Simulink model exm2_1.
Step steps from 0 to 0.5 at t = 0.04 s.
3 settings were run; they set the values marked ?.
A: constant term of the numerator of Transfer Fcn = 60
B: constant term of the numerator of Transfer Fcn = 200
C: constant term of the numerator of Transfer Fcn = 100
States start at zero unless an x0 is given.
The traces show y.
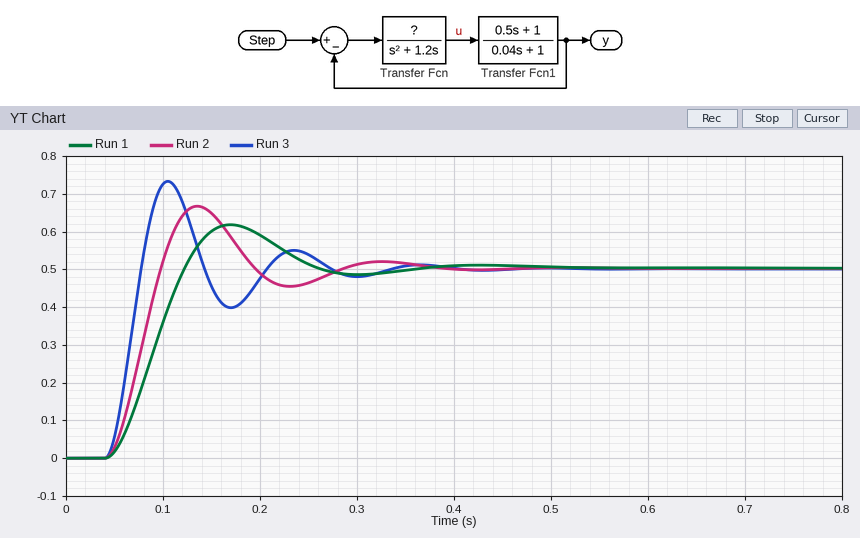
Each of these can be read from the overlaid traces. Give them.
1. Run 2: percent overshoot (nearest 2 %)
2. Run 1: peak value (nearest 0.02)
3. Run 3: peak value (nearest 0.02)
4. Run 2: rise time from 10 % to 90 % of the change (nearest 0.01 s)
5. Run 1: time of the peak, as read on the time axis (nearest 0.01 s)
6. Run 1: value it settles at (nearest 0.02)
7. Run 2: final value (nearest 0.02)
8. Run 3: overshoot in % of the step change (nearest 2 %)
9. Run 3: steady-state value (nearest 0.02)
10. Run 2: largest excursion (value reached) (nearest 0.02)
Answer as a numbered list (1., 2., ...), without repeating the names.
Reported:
1. 34 %
2. 0.62
3. 0.74
4. 0.04 s
5. 0.17 s
6. 0.50
7. 0.50
8. 46 %
9. 0.50
10. 0.66
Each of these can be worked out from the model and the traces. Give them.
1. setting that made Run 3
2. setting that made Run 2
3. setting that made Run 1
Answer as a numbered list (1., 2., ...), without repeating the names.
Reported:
1. B
2. C
3. A
